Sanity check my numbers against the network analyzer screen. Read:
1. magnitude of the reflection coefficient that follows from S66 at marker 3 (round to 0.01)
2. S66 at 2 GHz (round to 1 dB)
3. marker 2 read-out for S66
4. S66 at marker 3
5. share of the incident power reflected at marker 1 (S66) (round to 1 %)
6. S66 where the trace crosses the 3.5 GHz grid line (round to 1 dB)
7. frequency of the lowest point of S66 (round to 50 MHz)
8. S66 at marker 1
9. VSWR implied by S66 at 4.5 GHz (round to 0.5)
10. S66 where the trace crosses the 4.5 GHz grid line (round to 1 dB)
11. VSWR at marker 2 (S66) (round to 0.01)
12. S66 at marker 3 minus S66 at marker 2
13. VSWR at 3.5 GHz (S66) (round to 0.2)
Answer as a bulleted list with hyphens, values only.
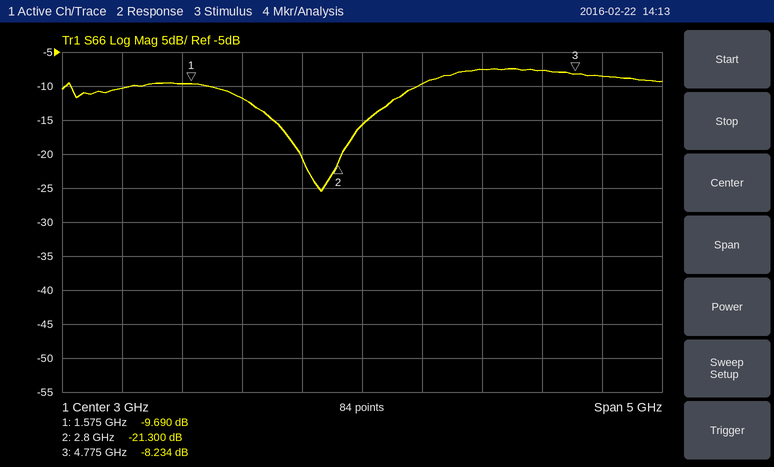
- 0.39
- -12 dB
- -21.300 dB
- -8.234 dB
- 11 %
- -10 dB
- 2.65 GHz
- -9.690 dB
- 2.5
- -8 dB
- 1.19
- 13.066 dB
- 2.0
